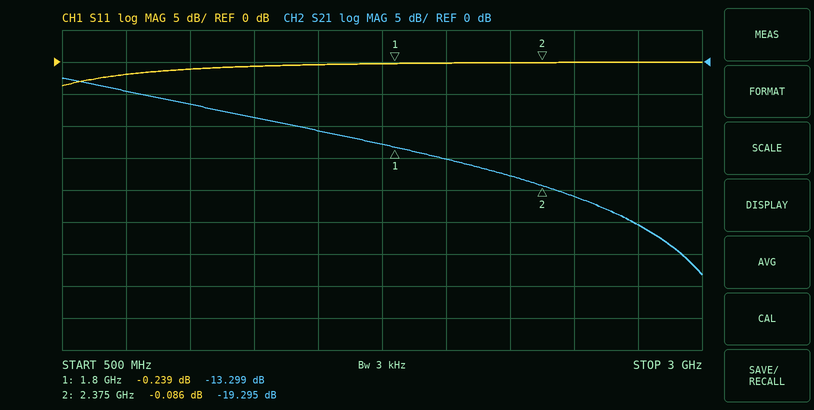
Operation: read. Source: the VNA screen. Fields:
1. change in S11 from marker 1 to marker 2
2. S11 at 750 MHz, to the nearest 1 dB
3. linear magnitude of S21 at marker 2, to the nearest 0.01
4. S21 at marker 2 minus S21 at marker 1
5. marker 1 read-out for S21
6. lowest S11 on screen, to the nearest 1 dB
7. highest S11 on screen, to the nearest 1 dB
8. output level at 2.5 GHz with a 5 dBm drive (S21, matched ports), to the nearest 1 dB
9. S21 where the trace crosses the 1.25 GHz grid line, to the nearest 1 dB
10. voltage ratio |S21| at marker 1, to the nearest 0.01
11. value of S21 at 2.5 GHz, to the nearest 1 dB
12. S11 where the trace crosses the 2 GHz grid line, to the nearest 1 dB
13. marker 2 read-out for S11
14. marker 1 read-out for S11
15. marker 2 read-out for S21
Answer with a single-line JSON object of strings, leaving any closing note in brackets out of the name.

{"change in S11 from marker 1 to marker 2": "0.153 dB", "S11 at 750 MHz, to the nearest 1 dB": "-2 dB", "linear magnitude of S21 at marker 2, to the nearest 0.01": "0.11", "S21 at marker 2 minus S21 at marker 1": "-5.996 dB", "marker 1 read-out for S21": "-13.299 dB", "lowest S11 on screen, to the nearest 1 dB": "-4 dB", "highest S11 on screen, to the nearest 1 dB": "0 dB", "output level at 2.5 GHz with a 5 dBm drive (S21, matched ports), to the nearest 1 dB": "-16 dBm", "S21 where the trace crosses the 1.25 GHz grid line, to the nearest 1 dB": "-9 dB", "voltage ratio |S21| at marker 1, to the nearest 0.01": "0.22", "value of S21 at 2.5 GHz, to the nearest 1 dB": "-21 dB", "S11 where the trace crosses the 2 GHz grid line, to the nearest 1 dB": "0 dB", "marker 2 read-out for S11": "-0.086 dB", "marker 1 read-out for S11": "-0.239 dB", "marker 2 read-out for S21": "-19.295 dB"}
